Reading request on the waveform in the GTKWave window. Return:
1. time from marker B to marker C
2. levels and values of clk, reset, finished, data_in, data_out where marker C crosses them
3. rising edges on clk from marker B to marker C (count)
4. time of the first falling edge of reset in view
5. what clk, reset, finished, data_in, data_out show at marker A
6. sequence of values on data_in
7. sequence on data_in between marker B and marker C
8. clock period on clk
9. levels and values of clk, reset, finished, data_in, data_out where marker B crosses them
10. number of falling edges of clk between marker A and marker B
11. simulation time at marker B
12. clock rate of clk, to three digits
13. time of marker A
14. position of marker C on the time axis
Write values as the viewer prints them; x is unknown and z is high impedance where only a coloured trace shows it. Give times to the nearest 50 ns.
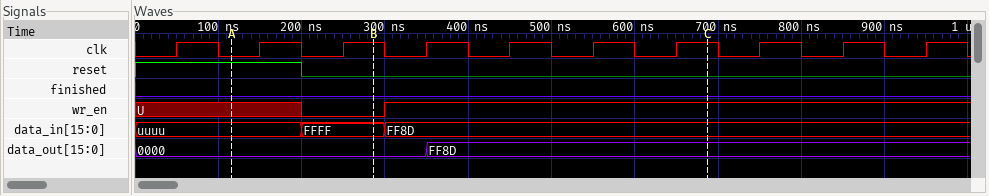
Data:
400 ns
clk=1, reset=0, finished=0, data_in=FF8D, data_out=FF8D
4
200 ns
clk=0, reset=1, finished=0, data_in=uuuu, data_out=0000
uuuu, FFFF, FF8D
FFFF, FF8D
100 ns
clk=1, reset=0, finished=0, data_in=FFFF, data_out=0000
1
300 ns
10.0 MHz
100 ns
700 ns
